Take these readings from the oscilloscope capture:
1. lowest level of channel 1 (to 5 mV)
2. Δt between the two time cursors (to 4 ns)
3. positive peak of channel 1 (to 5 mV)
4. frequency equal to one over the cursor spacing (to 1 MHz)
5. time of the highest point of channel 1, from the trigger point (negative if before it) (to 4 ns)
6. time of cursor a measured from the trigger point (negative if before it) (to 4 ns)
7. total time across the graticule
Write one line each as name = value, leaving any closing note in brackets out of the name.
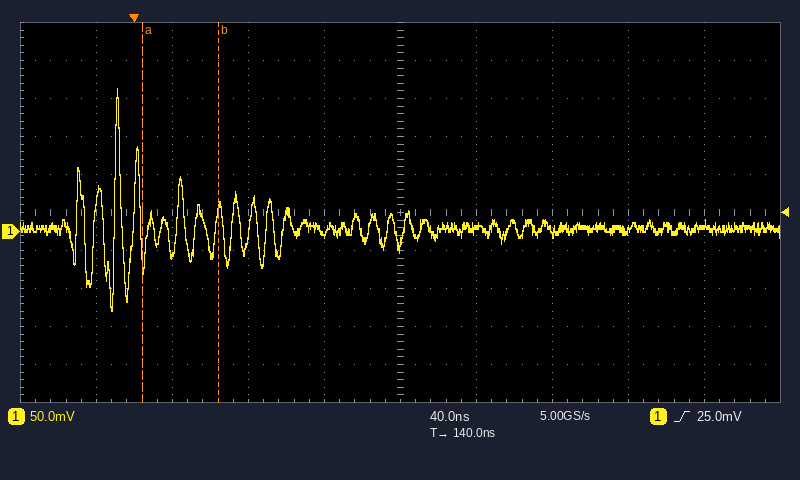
lowest level of channel 1 = -105 mV
Δt between the two time cursors = 40 ns
positive peak of channel 1 = 190 mV
frequency equal to one over the cursor spacing = 25 MHz
time of the highest point of channel 1, from the trigger point (negative if before it) = -8 ns
time of cursor a measured from the trigger point (negative if before it) = +4 ns
total time across the graticule = 400 ns
